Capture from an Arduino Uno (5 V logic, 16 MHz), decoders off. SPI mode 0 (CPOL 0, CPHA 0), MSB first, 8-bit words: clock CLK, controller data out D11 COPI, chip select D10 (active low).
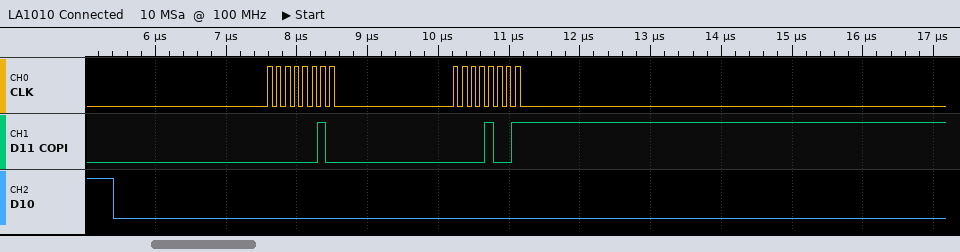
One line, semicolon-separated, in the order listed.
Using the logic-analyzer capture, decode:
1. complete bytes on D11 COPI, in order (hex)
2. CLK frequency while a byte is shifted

0x02 0x09; 8 MHz
